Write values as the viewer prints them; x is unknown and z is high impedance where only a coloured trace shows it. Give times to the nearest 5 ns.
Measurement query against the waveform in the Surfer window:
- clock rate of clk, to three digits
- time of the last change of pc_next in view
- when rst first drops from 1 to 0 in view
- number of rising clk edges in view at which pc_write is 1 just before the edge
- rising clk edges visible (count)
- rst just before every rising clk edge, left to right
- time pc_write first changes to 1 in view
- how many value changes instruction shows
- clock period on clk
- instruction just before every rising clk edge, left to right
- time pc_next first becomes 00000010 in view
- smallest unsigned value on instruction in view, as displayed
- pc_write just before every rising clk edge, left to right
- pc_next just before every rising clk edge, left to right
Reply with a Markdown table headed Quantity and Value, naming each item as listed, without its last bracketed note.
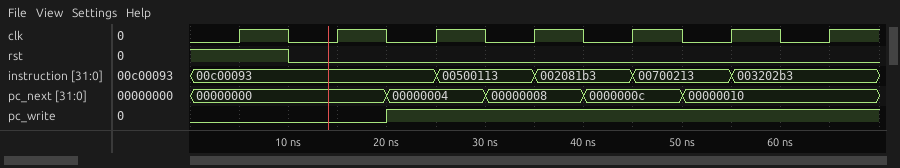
| Quantity | Value |
|---|---|
| clock rate of clk, to three digits | 100 MHz |
| time of the last change of pc_next in view | 50 ns |
| when rst first drops from 1 to 0 in view | 10 ns |
| number of rising clk edges in view at which pc_write is 1 just before the edge | 5 |
| rising clk edges visible | 7 |
| rst just before every rising clk edge, left to right | 1 0 0 0 0 0 0 |
| time pc_write first changes to 1 in view | 20 ns |
| how many value changes instruction shows | 4 |
| clock period on clk | 10 ns |
| instruction just before every rising clk edge, left to right | 00c00093, 00c00093, 00c00093, 00500113, 002081b3, 00700213, 003202b3 |
| time pc_next first becomes 00000010 in view | 50 ns |
| smallest unsigned value on instruction in view, as displayed | 002081b3 |
| pc_write just before every rising clk edge, left to right | 0 0 1 1 1 1 1 |
| pc_next just before every rising clk edge, left to right | 00000000, 00000000, 00000004, 00000008, 0000000c, 00000010, 00000010 |
